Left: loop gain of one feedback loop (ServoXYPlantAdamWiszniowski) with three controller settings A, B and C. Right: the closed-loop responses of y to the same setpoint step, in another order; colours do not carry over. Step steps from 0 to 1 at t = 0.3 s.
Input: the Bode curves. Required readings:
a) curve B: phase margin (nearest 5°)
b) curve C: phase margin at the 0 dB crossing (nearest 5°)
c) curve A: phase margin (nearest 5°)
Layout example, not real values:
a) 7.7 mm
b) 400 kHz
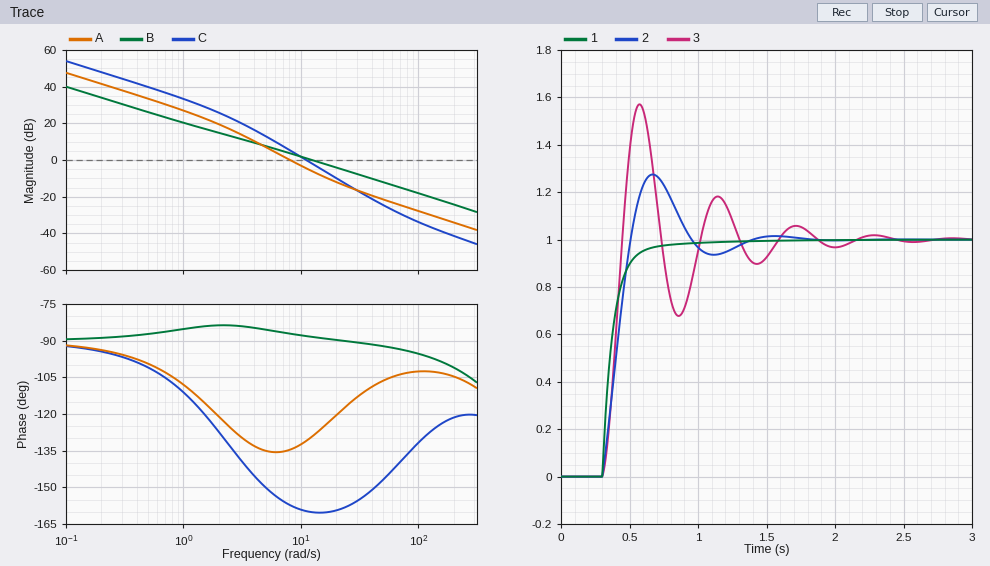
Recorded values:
a) 90°
b) 20°
c) 45°
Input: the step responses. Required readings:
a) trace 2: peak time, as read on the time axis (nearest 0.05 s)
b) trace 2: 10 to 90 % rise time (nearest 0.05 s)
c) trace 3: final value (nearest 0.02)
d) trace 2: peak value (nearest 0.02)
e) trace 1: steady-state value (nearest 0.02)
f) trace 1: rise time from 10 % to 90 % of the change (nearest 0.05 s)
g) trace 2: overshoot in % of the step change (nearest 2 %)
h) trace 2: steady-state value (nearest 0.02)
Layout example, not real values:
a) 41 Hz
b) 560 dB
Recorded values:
a) 0.65 s
b) 0.15 s
c) 1.00
d) 1.28
e) 1.00
f) 0.20 s
g) 28 %
h) 1.00
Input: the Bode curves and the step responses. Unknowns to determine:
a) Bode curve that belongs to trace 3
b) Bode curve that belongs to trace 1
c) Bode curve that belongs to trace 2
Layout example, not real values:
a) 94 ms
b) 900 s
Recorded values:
a) C
b) B
c) A
